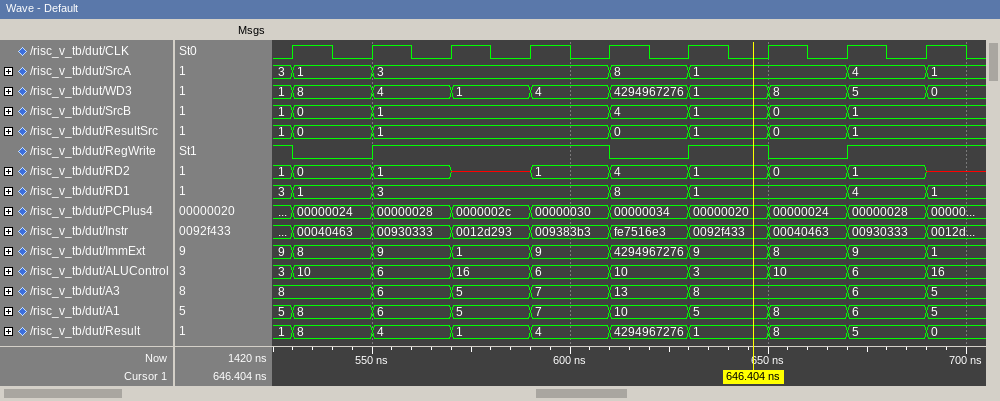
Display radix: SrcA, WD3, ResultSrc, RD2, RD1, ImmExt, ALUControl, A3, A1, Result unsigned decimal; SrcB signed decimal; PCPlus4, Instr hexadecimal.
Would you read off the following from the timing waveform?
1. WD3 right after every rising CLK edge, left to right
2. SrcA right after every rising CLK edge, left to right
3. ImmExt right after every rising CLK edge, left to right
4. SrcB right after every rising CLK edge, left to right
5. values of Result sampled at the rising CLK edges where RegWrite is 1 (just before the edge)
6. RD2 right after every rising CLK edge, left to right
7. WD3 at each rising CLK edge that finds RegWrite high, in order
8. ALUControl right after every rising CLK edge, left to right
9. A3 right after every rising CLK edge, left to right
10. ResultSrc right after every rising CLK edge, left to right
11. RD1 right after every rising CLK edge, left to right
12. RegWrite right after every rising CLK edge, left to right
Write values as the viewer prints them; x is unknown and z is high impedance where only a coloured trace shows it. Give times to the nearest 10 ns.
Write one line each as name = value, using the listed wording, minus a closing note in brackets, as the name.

WD3 right after every rising CLK edge, left to right = 8, 4, 1, 4, 4294967276, 1, 8, 5, 0
SrcA right after every rising CLK edge, left to right = 1, 3, 3, 3, 8, 1, 1, 4, 1
ImmExt right after every rising CLK edge, left to right = 8, 9, 1, 9, 4294967276, 9, 8, 9, 1
SrcB right after every rising CLK edge, left to right = 0, 1, 1, 1, 4, 1, 0, 1, 1
values of Result sampled at the rising CLK edges where RegWrite is 1 = 1, 4, 1, 4, 1, 5
RD2 right after every rising CLK edge, left to right = 0, 1, x, 1, 4, 1, 0, 1, x
WD3 at each rising CLK edge that finds RegWrite high, in order = 1, 4, 1, 4, 1, 5
ALUControl right after every rising CLK edge, left to right = 10, 6, 16, 6, 10, 3, 10, 6, 16
A3 right after every rising CLK edge, left to right = 8, 6, 5, 7, 13, 8, 8, 6, 5
ResultSrc right after every rising CLK edge, left to right = 0, 1, 1, 1, 0, 1, 0, 1, 1
RD1 right after every rising CLK edge, left to right = 1, 3, 3, 3, 8, 1, 1, 4, 1
RegWrite right after every rising CLK edge, left to right = 0 1 1 1 0 1 0 1 1
